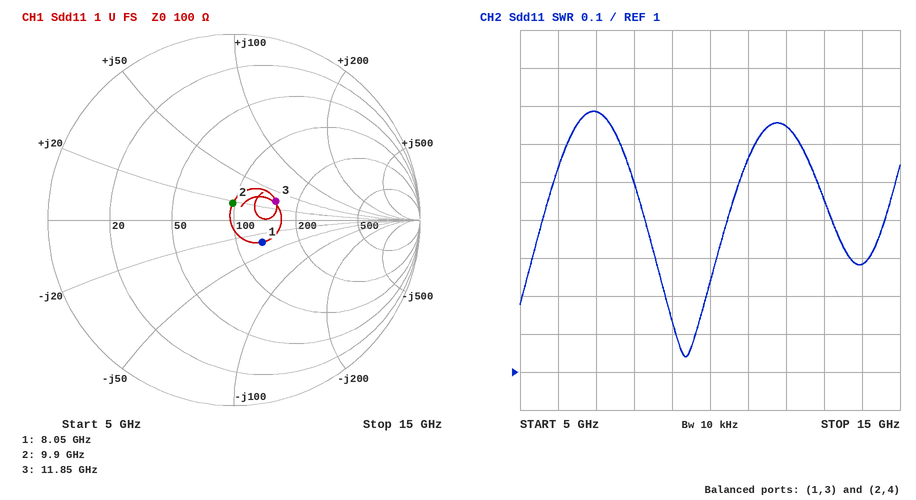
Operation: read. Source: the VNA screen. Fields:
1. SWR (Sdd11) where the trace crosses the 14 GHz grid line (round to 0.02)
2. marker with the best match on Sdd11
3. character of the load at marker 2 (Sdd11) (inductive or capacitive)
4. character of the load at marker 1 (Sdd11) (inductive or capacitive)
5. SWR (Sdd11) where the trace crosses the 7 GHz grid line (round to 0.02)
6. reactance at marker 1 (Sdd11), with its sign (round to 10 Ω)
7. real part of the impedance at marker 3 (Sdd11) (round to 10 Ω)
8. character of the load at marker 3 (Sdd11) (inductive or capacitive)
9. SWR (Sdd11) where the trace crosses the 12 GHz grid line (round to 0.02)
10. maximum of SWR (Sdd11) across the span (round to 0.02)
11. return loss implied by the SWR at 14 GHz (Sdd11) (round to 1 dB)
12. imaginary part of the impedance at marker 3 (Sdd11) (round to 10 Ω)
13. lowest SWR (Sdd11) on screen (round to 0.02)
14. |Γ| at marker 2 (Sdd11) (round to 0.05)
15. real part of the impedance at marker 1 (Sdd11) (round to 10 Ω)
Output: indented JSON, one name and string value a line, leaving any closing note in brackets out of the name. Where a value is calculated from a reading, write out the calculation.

{
  "SWR (Sdd11) where the trace crosses the 14 GHz grid line": "1.28",
  "marker with the best match on Sdd11": "marker 2",
  "character of the load at marker 2 (Sdd11)": "inductive",
  "character of the load at marker 1 (Sdd11)": "capacitive",
  "SWR (Sdd11) where the trace crosses the 7 GHz grid line": "1.68",
  "reactance at marker 1 (Sdd11), with its sign": "-30 Ω",
  "real part of the impedance at marker 3 (Sdd11)": "150 Ω",
  "character of the load at marker 3 (Sdd11)": "inductive",
  "SWR (Sdd11) where the trace crosses the 12 GHz grid line": "1.64",
  "maximum of SWR (Sdd11) across the span": "1.68",
  "return loss implied by the SWR at 14 GHz (Sdd11)": "−20 log10((1.28 − 1)/(1.28 + 1)) ≈ 18 dB",
  "imaginary part of the impedance at marker 3 (Sdd11)": "+30 Ω",
  "lowest SWR (Sdd11) on screen": "1.04",
  "|Γ| at marker 2 (Sdd11)": "0.10",
  "real part of the impedance at marker 1 (Sdd11)": "130 Ω"
}
